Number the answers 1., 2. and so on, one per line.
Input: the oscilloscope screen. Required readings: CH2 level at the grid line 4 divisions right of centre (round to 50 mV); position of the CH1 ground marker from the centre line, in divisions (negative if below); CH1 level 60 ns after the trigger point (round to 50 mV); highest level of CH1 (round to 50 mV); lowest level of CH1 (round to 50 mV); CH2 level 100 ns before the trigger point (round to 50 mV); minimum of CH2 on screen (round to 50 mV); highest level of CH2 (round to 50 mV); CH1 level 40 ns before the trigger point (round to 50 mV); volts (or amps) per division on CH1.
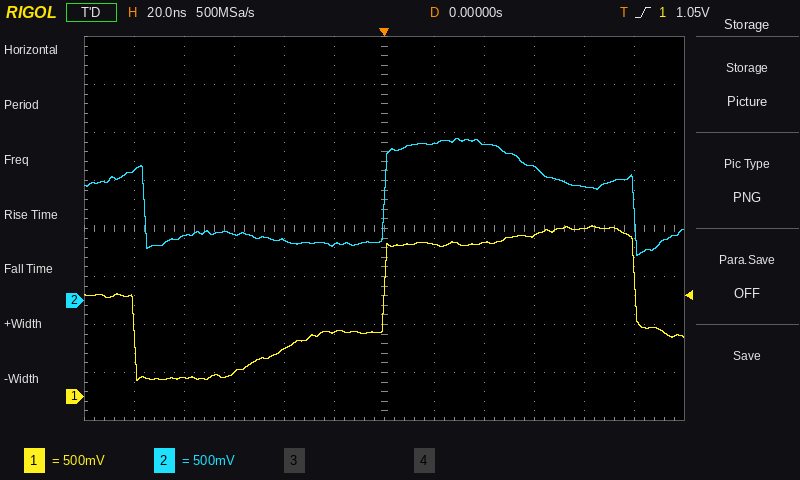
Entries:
1. 1.20 V
2. -3.5 div
3. 1.70 V
4. 1.80 V
5. 150 mV
6. 1.35 V
7. 450 mV
8. 1.70 V
9. 500 mV
10. 500 mV
